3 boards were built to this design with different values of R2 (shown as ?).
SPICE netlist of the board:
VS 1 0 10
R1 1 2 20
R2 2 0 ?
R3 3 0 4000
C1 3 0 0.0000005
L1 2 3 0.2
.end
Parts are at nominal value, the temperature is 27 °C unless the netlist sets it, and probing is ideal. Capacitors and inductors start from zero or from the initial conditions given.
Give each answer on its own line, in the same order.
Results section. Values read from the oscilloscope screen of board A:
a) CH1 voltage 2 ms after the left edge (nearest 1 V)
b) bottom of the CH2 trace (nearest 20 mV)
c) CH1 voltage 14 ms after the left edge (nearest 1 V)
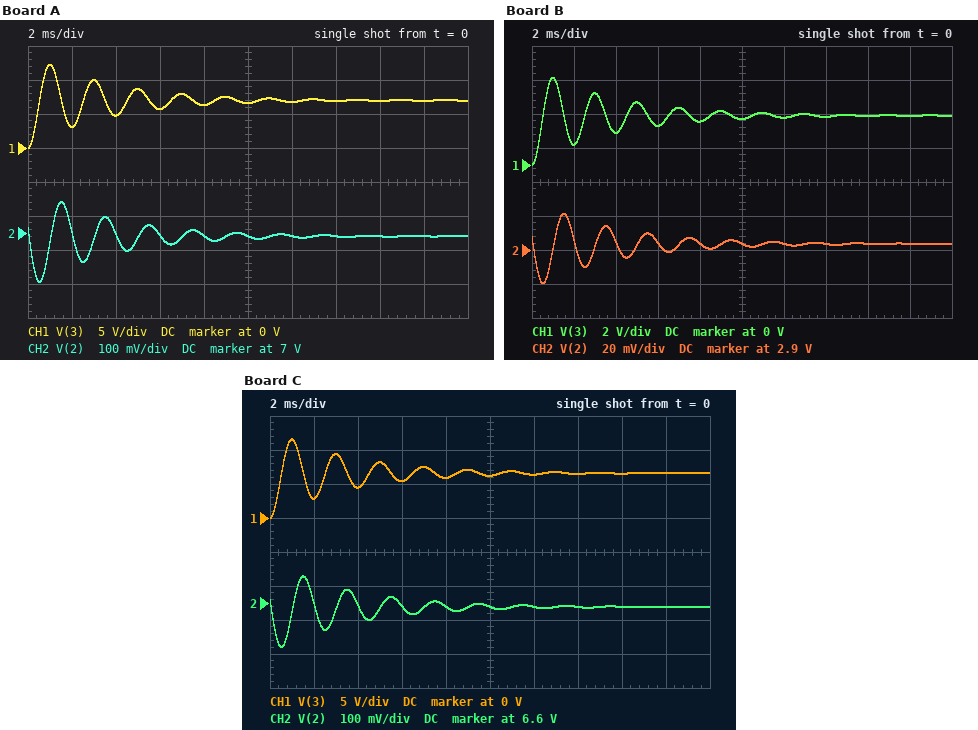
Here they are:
3 V
6.86 V
7 V
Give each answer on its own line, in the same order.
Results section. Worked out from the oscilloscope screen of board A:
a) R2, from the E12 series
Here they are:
47 Ω
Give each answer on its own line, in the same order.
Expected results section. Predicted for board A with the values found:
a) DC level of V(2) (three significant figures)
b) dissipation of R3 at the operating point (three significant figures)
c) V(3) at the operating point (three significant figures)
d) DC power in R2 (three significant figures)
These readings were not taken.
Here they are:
6.99 V
12.2 mW
6.99 V
1.04 W
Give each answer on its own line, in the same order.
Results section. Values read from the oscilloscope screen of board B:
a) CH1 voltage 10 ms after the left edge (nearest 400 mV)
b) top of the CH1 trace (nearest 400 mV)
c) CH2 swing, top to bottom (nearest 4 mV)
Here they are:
2.8 V
5.2 V
40 mV
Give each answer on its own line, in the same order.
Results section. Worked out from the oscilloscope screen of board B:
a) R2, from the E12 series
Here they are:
8.2 Ω
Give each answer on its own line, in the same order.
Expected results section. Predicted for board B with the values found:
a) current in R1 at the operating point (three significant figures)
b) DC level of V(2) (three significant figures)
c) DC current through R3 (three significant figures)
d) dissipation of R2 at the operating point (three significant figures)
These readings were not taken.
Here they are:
355 mA
2.90 V
726 µA
1.03 W
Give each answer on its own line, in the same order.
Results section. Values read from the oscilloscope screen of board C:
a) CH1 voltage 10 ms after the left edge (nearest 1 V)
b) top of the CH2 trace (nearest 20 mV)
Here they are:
6 V
6.68 V
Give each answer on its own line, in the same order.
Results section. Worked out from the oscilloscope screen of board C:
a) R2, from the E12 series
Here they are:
39 Ω
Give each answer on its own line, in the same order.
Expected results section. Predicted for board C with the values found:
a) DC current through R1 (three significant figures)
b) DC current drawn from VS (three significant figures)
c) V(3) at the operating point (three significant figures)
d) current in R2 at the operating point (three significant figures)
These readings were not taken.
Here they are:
171 mA
171 mA
6.59 V
169 mA
